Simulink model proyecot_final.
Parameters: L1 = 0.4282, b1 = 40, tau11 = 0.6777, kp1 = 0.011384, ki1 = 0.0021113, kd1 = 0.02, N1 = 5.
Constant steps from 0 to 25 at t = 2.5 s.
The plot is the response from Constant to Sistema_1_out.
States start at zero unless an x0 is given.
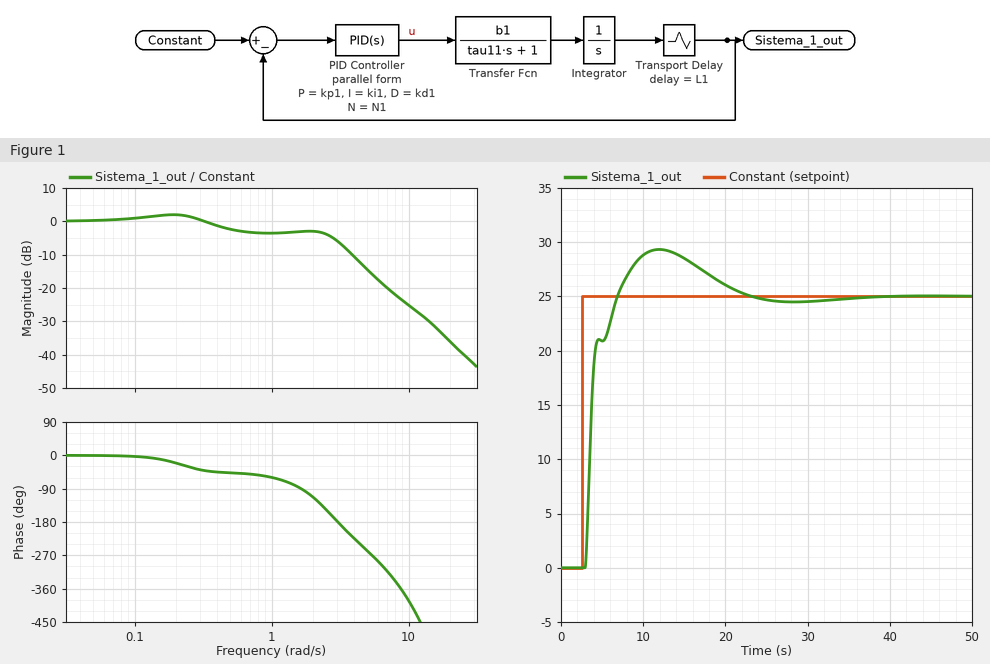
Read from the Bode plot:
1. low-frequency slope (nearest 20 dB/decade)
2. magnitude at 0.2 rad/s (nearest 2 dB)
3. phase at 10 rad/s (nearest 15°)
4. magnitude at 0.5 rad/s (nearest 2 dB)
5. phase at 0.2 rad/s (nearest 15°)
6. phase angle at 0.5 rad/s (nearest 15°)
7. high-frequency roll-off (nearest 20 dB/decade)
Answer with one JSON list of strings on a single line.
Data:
["0 dB/decade", "2 dB", "-390°", "-2 dB", "-15°", "-45°", "-40 dB/decade"]
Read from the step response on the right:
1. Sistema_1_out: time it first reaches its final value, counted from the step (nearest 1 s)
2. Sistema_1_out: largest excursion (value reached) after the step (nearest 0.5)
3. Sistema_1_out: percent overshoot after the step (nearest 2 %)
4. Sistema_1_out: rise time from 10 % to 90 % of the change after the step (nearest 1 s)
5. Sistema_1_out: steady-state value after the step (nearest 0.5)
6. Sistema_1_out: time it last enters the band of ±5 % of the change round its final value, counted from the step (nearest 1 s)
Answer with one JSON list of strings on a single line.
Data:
["4 s", "29.5", "18 %", "3 s", "25.0", "17 s"]
